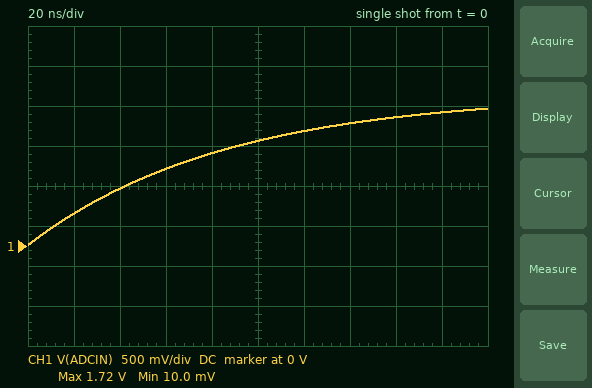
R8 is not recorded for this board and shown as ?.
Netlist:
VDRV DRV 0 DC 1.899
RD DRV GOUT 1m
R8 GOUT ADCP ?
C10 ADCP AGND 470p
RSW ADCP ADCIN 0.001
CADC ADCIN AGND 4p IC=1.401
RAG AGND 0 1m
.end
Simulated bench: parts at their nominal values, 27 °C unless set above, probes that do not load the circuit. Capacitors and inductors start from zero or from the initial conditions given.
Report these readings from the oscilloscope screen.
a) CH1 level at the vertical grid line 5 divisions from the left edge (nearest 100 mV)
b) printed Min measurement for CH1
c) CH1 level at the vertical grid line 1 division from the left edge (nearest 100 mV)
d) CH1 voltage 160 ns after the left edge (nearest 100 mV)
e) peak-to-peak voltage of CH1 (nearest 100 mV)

1.3 V
10.0 mV
400 mV
1.6 V
1.7 V
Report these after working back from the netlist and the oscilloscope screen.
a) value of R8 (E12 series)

180 Ω
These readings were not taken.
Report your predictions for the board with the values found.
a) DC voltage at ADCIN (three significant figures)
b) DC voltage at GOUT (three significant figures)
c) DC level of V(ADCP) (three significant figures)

1.90 V
1.90 V
1.90 V
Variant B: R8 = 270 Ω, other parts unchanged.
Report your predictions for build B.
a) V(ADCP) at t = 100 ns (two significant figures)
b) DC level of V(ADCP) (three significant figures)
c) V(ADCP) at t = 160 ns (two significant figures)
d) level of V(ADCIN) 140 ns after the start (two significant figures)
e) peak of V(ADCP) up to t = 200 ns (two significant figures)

1.0 V
1.90 V
1.4 V
1.3 V
1.5 V
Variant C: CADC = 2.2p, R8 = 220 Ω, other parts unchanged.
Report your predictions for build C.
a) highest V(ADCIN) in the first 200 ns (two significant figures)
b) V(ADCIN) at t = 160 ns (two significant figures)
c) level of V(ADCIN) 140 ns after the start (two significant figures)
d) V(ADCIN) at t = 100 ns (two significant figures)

1.6 V
1.5 V
1.4 V
1.2 V
